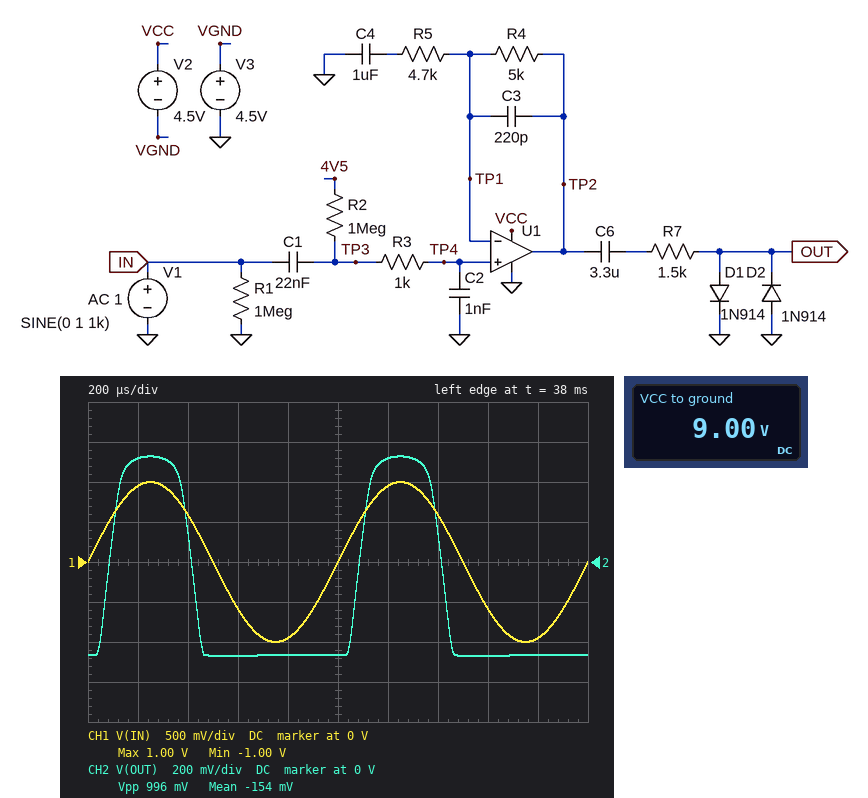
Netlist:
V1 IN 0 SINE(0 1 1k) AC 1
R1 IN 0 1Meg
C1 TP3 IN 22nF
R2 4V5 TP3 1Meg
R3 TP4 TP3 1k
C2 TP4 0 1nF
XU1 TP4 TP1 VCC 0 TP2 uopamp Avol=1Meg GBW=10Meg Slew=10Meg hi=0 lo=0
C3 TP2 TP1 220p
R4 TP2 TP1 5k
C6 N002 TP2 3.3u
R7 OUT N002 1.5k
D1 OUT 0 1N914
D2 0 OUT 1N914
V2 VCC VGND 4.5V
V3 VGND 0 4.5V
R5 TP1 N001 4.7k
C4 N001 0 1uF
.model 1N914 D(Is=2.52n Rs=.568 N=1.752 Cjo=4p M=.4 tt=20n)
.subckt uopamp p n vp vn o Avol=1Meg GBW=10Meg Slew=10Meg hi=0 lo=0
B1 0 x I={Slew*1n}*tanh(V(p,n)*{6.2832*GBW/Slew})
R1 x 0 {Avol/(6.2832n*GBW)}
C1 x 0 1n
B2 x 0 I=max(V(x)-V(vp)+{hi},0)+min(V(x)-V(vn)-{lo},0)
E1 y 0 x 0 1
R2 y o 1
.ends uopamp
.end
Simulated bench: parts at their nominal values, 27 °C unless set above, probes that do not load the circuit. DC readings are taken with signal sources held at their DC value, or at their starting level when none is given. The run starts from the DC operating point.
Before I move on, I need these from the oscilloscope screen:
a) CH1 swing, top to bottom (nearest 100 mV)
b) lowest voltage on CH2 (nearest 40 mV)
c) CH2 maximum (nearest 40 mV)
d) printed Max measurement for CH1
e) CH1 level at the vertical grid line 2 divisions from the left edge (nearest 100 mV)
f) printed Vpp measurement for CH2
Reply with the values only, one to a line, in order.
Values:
2.0 V
-480 mV
520 mV
1.00 V
600 mV
996 mV
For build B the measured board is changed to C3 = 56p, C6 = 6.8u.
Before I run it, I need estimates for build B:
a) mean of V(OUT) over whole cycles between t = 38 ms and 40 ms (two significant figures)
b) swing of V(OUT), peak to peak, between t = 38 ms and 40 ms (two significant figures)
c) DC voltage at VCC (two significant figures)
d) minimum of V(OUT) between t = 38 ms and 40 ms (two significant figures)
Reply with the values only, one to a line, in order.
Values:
-130 mV
980 mV
9.0 V
-450 mV
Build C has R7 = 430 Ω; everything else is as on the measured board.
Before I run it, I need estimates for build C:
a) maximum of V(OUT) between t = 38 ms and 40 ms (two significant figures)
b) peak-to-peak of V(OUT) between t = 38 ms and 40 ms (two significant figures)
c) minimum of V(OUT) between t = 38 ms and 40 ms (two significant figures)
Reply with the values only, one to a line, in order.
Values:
580 mV
1.1 V
-520 mV
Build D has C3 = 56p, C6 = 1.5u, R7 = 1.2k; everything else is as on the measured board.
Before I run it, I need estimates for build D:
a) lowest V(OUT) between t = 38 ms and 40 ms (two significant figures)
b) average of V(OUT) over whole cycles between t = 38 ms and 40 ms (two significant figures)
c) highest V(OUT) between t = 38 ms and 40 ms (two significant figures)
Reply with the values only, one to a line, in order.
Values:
-480 mV
-160 mV
540 mV
